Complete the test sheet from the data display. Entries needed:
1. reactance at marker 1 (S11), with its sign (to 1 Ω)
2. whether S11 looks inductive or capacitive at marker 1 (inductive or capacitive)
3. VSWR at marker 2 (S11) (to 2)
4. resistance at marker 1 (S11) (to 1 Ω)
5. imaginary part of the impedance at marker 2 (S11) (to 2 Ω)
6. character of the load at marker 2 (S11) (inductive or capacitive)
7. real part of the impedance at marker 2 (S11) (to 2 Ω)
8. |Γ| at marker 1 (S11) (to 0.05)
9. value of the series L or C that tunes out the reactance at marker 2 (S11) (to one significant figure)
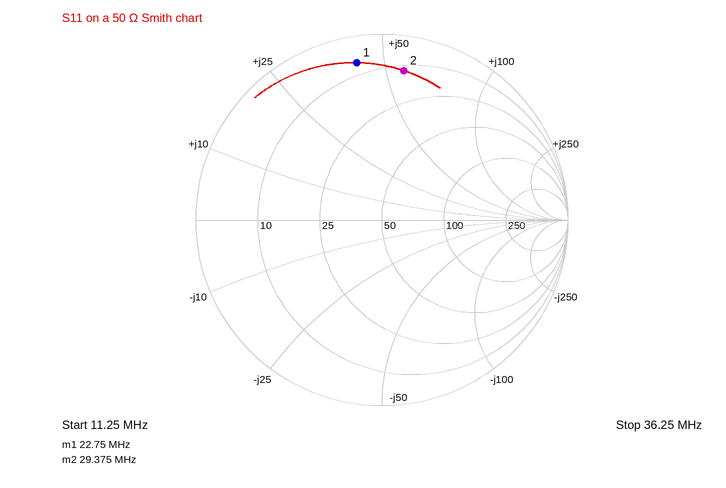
+42 Ω
inductive
10
7 Ω
+56 Ω
inductive
12 Ω
0.85
100 pF
